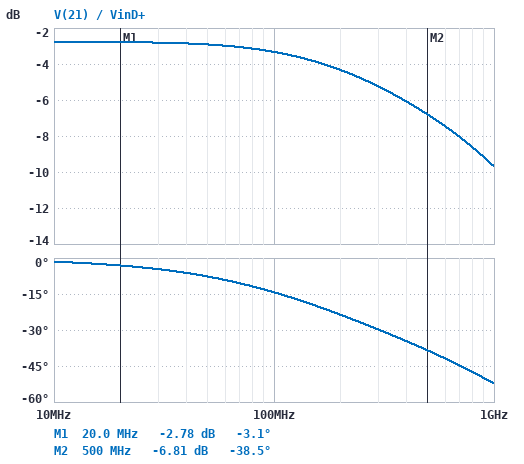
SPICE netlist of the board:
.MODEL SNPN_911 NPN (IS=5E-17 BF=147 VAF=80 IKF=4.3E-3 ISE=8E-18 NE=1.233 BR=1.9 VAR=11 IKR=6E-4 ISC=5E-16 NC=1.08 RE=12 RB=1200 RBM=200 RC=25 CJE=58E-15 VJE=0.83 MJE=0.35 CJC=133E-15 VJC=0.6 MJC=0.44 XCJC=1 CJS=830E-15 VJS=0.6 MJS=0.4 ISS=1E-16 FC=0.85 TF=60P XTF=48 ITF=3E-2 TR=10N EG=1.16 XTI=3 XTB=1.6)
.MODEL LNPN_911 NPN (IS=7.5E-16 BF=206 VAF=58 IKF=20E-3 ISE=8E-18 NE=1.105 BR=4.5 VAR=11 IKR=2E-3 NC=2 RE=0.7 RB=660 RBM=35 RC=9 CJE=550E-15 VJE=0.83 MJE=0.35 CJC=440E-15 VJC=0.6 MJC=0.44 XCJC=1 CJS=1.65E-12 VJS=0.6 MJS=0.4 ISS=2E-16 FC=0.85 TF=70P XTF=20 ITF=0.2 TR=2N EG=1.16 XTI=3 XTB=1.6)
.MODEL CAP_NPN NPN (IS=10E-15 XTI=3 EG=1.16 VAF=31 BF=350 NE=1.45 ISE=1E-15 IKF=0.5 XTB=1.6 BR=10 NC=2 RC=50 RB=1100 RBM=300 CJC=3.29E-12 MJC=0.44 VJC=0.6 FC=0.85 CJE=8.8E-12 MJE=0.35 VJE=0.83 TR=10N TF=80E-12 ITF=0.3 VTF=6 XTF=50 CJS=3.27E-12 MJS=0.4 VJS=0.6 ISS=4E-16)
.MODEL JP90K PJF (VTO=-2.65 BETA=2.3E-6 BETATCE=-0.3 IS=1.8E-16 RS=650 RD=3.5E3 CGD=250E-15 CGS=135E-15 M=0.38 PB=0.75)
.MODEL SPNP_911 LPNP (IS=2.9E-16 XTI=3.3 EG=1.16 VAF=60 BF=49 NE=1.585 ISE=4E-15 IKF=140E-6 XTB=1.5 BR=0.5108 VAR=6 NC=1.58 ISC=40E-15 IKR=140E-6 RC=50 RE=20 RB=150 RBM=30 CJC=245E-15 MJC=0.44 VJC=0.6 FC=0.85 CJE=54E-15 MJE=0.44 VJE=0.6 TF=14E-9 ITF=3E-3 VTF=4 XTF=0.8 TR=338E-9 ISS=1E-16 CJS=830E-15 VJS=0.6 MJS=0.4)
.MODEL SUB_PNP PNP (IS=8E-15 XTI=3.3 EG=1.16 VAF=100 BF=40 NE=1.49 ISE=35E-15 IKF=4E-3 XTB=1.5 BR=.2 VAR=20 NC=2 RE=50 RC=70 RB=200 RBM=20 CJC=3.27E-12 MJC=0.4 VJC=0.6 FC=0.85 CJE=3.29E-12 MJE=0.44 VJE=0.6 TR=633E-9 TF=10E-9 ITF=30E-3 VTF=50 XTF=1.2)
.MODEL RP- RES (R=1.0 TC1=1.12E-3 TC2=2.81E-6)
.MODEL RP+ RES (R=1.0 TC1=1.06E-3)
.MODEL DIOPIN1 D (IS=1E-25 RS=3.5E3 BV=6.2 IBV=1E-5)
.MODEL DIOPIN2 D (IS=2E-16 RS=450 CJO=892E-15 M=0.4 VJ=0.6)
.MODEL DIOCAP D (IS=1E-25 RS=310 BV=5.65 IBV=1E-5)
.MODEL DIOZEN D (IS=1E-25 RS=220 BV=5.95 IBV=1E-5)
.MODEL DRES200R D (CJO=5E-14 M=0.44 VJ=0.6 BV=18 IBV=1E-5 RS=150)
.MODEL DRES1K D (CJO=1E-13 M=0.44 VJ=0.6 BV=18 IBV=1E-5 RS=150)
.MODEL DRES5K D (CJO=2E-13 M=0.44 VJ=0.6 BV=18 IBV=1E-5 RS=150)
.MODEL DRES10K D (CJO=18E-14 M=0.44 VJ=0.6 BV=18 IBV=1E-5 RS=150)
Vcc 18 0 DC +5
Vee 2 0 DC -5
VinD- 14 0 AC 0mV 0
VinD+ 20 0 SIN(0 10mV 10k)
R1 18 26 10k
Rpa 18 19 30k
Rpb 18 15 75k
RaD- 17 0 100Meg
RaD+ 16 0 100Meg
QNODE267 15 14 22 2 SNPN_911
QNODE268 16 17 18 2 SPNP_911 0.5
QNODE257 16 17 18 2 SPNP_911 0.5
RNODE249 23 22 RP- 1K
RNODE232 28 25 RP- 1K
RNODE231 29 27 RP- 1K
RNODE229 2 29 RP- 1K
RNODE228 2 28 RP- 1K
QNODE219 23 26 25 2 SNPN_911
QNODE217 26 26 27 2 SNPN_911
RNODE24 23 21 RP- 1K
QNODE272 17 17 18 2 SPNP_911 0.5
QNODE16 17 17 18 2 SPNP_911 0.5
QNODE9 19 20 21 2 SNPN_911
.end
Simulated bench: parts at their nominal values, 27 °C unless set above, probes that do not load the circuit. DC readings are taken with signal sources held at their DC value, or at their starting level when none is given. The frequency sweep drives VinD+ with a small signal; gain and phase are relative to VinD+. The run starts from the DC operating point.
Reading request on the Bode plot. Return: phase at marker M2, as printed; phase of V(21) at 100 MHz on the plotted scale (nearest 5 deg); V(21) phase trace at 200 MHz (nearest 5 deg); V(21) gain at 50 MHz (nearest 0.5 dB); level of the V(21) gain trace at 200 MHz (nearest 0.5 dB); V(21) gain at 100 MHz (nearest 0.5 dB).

-38.5 deg
-15 deg
-25 deg
-3.0 dB
-4.5 dB
-3.5 dB
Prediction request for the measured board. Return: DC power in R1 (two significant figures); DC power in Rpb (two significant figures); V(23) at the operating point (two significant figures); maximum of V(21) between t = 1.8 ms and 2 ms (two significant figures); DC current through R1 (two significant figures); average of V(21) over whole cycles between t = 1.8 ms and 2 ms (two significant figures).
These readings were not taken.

5.9 mW
480 µW
-1.4 V
-970 mV
770 µA
-980 mV
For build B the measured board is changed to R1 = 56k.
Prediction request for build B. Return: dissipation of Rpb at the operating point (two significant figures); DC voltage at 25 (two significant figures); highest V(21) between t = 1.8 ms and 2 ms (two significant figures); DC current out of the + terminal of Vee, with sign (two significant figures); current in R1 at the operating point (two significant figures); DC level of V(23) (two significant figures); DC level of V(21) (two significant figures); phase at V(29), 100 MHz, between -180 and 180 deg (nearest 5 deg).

420 µW
-4.7 V
-720 mV
-320 µA
160 µA
-810 mV
-730 mV
25 deg
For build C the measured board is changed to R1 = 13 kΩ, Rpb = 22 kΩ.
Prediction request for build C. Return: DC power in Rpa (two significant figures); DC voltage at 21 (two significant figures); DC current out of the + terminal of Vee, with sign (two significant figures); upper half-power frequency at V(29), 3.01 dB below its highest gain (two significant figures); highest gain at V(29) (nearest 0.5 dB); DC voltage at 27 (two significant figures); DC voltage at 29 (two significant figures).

1.1 mW
-860 mV
-1.2 mA
410 MHz
-36.0 dB
-3.8 V
-4.4 V
